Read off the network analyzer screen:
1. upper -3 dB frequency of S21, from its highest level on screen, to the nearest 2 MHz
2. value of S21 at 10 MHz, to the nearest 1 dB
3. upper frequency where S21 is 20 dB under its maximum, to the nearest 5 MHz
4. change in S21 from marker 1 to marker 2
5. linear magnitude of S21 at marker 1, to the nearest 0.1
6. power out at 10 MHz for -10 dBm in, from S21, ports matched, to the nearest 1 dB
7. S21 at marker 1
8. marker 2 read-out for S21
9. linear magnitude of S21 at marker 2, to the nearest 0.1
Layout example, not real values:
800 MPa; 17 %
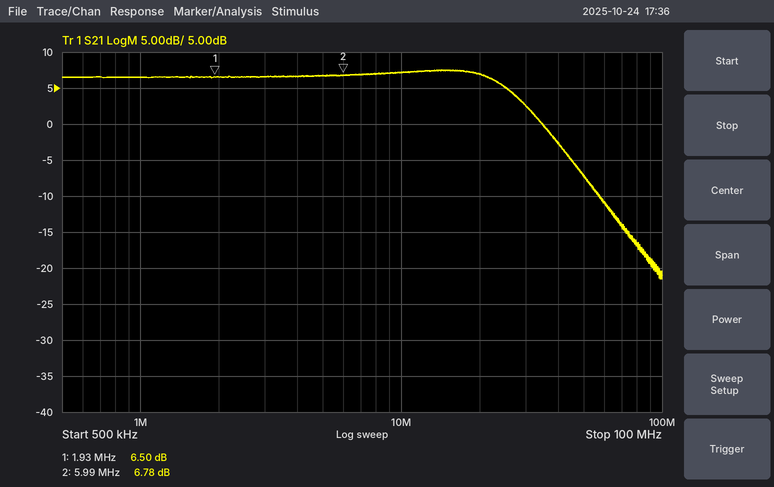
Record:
26 MHz; 7 dB; 65 MHz; 0.28 dB; 2.1; -3 dBm; 6.50 dB; 6.78 dB; 2.2
